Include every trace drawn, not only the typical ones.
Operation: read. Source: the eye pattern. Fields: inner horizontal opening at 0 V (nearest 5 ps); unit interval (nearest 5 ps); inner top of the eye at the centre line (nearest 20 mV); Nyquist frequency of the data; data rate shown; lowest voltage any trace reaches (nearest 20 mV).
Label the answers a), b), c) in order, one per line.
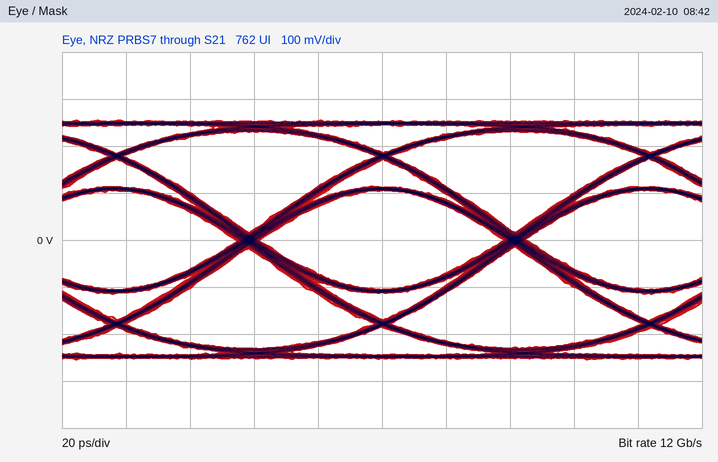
a) 75 ps
b) 85 ps
c) 100 mV
d) 6 GHz
e) 12 Gb/s
f) -260 mV
